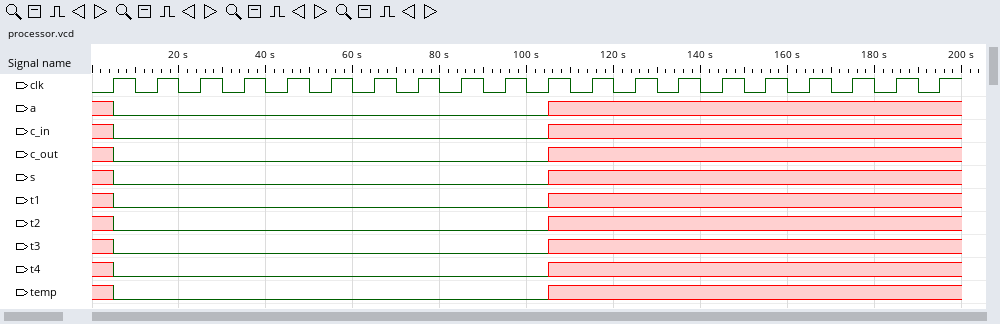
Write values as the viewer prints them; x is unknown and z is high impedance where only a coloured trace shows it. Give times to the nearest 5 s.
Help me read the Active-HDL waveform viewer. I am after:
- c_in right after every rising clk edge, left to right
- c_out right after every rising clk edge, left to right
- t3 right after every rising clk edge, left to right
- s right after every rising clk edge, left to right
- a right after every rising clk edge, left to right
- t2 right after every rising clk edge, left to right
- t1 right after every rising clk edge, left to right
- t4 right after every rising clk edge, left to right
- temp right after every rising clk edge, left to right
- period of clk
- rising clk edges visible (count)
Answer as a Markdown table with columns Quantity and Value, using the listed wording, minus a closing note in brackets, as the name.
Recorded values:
| Quantity | Value |
|---|---|
| c_in right after every rising clk edge, left to right | 0 0 0 0 0 0 0 0 0 0 x x x x x x x x x x |
| c_out right after every rising clk edge, left to right | 0 0 0 0 0 0 0 0 0 0 x x x x x x x x x x |
| t3 right after every rising clk edge, left to right | 0 0 0 0 0 0 0 0 0 0 x x x x x x x x x x |
| s right after every rising clk edge, left to right | 0 0 0 0 0 0 0 0 0 0 x x x x x x x x x x |
| a right after every rising clk edge, left to right | 0 0 0 0 0 0 0 0 0 0 x x x x x x x x x x |
| t2 right after every rising clk edge, left to right | 0 0 0 0 0 0 0 0 0 0 x x x x x x x x x x |
| t1 right after every rising clk edge, left to right | 0 0 0 0 0 0 0 0 0 0 x x x x x x x x x x |
| t4 right after every rising clk edge, left to right | 0 0 0 0 0 0 0 0 0 0 x x x x x x x x x x |
| temp right after every rising clk edge, left to right | 0 0 0 0 0 0 0 0 0 0 x x x x x x x x x x |
| period of clk | 10 s |
| rising clk edges visible | 20 |
